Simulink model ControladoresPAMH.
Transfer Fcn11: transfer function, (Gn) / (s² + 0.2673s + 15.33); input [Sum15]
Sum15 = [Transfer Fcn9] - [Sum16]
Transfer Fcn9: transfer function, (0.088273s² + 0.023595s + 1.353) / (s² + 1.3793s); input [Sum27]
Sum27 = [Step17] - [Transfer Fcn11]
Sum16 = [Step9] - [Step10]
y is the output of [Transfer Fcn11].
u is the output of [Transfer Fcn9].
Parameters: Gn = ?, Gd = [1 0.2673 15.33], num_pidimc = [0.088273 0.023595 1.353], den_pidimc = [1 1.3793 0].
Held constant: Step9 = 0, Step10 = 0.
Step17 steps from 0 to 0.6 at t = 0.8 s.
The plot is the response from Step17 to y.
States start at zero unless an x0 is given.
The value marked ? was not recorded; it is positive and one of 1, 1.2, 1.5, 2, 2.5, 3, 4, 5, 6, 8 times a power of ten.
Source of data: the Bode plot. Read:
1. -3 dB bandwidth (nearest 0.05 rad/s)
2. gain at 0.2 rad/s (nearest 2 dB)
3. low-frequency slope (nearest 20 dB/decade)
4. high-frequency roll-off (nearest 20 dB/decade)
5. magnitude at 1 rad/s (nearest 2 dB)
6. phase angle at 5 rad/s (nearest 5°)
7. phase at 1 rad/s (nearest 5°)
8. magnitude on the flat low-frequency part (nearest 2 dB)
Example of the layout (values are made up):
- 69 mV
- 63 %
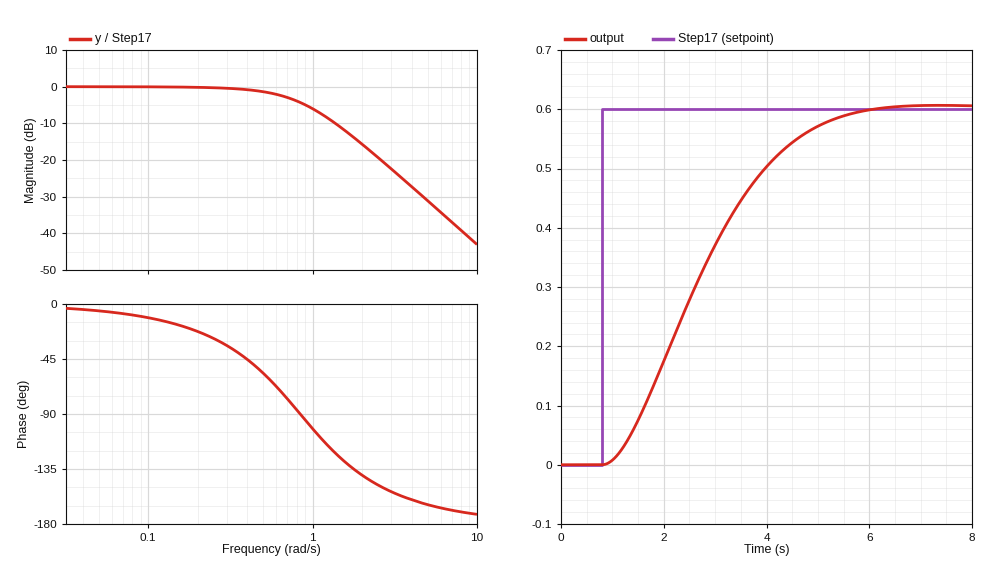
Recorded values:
- 0.70 rad/s
- 0 dB
- 0 dB/decade
- -40 dB/decade
- -6 dB
- -165°
- -100°
- 0 dB
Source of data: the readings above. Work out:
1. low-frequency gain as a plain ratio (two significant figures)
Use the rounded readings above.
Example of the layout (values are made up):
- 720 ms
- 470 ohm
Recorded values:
- 1.0
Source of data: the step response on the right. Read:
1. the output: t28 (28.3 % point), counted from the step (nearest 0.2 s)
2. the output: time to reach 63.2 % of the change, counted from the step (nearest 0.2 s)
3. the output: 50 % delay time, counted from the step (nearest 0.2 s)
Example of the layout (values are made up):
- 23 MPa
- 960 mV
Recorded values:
- 1.2 s
- 2.2 s
- 1.8 s
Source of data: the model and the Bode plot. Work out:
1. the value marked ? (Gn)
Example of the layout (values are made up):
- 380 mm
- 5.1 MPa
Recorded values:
- 8
